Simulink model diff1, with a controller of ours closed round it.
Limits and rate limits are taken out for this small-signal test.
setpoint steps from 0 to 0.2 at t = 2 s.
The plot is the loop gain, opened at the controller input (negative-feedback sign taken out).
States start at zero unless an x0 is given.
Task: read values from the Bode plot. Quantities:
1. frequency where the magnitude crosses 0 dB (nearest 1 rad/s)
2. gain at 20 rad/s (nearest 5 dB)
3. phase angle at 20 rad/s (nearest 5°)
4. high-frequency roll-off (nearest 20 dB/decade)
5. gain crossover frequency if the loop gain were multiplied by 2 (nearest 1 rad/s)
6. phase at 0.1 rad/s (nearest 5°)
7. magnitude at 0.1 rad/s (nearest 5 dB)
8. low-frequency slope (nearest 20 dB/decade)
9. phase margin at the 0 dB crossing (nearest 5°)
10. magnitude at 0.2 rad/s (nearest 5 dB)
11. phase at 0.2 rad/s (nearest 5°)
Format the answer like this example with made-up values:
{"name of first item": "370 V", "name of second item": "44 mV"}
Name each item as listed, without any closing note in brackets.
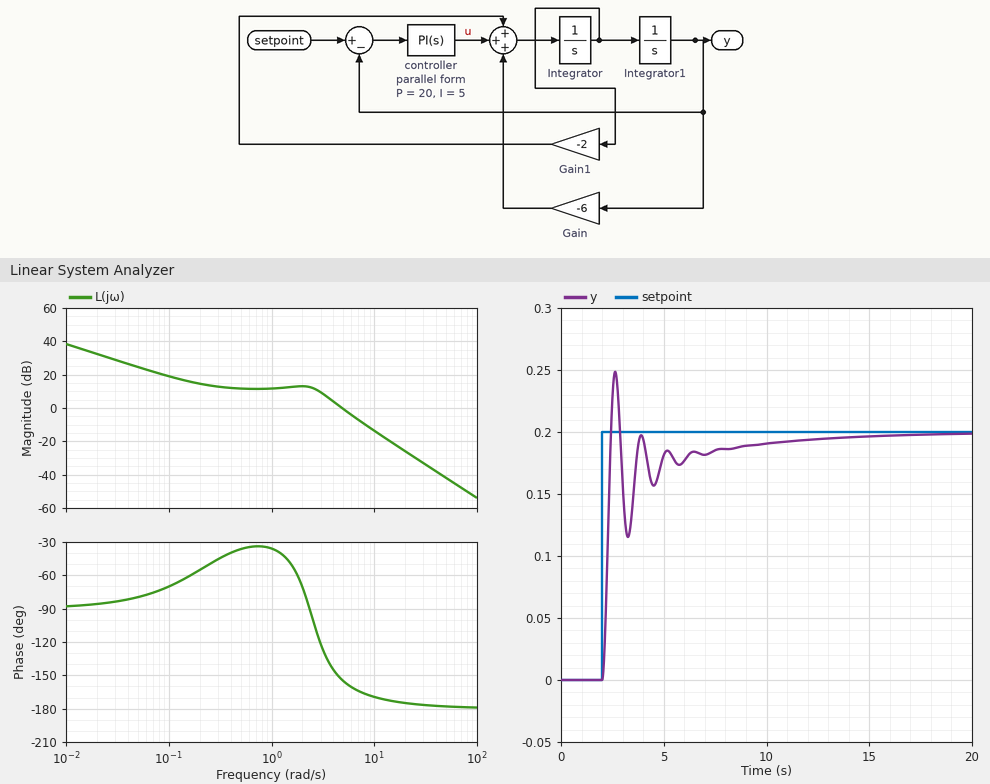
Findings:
{"frequency where the magnitude crosses 0 dB": "5 rad/s", "gain at 20 rad/s": "-25 dB", "phase angle at 20 rad/s": "-175°", "high-frequency roll-off": "-40 dB/decade", "gain crossover frequency if the loop gain were multiplied by 2": "7 rad/s", "phase at 0.1 rad/s": "-70°", "magnitude at 0.1 rad/s": "20 dB", "low-frequency slope": "-20 dB/decade", "phase margin at the 0 dB crossing": "25°", "magnitude at 0.2 rad/s": "15 dB", "phase at 0.2 rad/s": "-55°"}
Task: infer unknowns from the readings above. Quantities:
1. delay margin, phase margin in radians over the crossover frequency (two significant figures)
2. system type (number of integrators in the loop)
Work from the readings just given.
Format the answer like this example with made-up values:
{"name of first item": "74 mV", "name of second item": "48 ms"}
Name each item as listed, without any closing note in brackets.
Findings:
{"delay margin, phase margin in radians over the crossover frequency": "0.087 s", "system type": "1"}
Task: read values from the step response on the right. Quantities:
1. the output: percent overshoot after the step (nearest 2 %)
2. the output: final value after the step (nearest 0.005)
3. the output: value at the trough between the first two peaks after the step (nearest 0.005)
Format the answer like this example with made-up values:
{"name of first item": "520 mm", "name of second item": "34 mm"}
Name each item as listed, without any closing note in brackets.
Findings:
{"the output: percent overshoot after the step": "24 %", "the output: final value after the step": "0.200", "the output: value at the trough between the first two peaks after the step": "0.115"}
